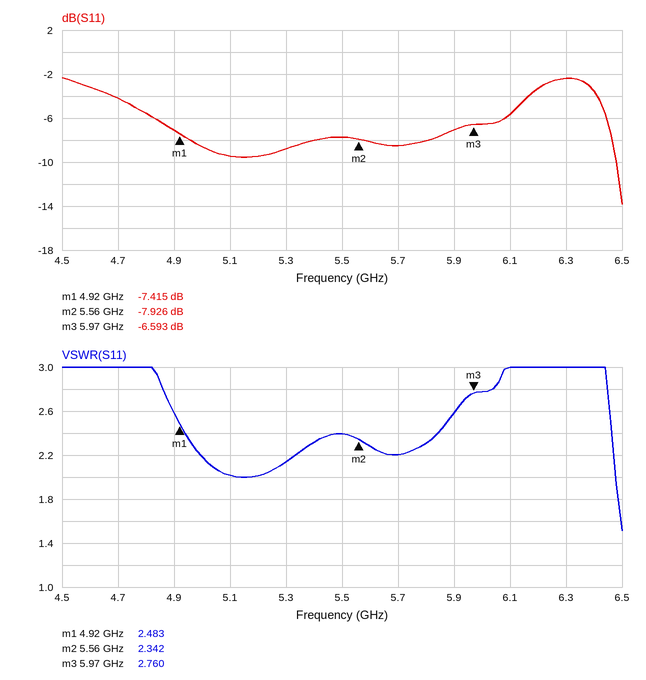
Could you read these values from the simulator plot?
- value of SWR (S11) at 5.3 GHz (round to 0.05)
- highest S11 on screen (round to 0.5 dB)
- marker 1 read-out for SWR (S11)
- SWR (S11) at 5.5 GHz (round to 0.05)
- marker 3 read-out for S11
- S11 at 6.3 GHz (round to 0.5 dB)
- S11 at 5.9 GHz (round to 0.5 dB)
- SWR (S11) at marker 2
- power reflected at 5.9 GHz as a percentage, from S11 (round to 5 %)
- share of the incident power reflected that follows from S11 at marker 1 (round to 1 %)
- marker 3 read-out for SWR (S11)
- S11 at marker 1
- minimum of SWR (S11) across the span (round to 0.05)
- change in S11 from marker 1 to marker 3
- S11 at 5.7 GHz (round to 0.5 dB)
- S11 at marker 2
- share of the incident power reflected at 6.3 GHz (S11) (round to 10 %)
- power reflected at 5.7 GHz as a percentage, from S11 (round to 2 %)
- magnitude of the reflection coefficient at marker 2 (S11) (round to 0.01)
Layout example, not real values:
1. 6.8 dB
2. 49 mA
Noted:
1. 2.15
2. -2.5 dB
3. 2.483
4. 2.40
5. -6.593 dB
6. -2.5 dB
7. -7.0 dB
8. 2.342
9. 20 %
10. 18 %
11. 2.760
12. -7.415 dB
13. 1.50
14. 0.822 dB
15. -8.5 dB
16. -7.926 dB
17. 60 %
18. 14 %
19. 0.40
